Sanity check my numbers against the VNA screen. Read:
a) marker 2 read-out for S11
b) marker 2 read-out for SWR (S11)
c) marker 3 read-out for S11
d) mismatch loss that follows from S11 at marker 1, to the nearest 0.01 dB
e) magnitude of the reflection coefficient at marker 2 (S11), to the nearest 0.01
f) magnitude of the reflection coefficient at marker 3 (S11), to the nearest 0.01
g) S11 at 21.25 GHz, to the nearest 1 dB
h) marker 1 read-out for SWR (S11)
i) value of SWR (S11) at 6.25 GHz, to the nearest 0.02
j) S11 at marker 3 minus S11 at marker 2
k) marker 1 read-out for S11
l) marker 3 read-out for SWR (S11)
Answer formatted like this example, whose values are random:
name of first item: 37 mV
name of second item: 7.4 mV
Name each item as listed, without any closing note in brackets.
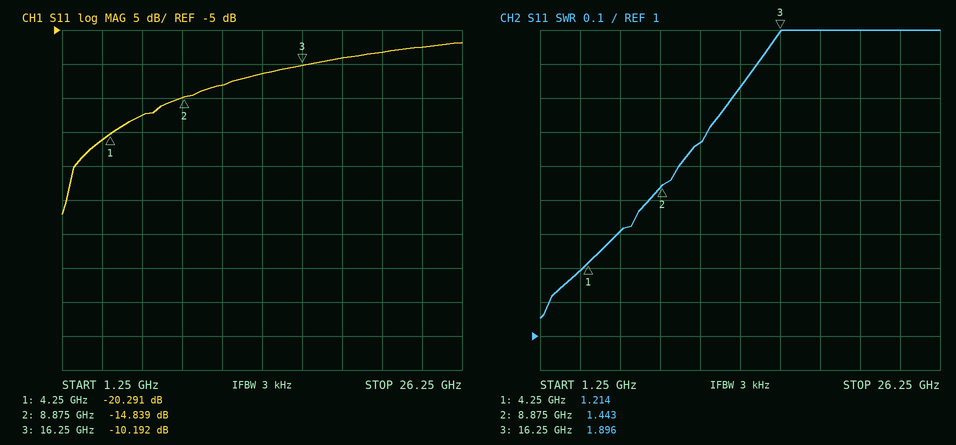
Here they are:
marker 2 read-out for S11: -14.839 dB
marker 2 read-out for SWR: 1.443
marker 3 read-out for S11: -10.192 dB
mismatch loss that follows from S11 at marker 1, to the nearest 0.01 dB: 0.04 dB
magnitude of the reflection coefficient at marker 2 (S11), to the nearest 0.01: 0.18
magnitude of the reflection coefficient at marker 3 (S11), to the nearest 0.01: 0.31
S11 at 21.25 GHz, to the nearest 1 dB: -8 dB
marker 1 read-out for SWR: 1.214
value of SWR (S11) at 6.25 GHz, to the nearest 0.02: 1.30
S11 at marker 3 minus S11 at marker 2: 4.647 dB
marker 1 read-out for S11: -20.291 dB
marker 3 read-out for SWR: 1.896
